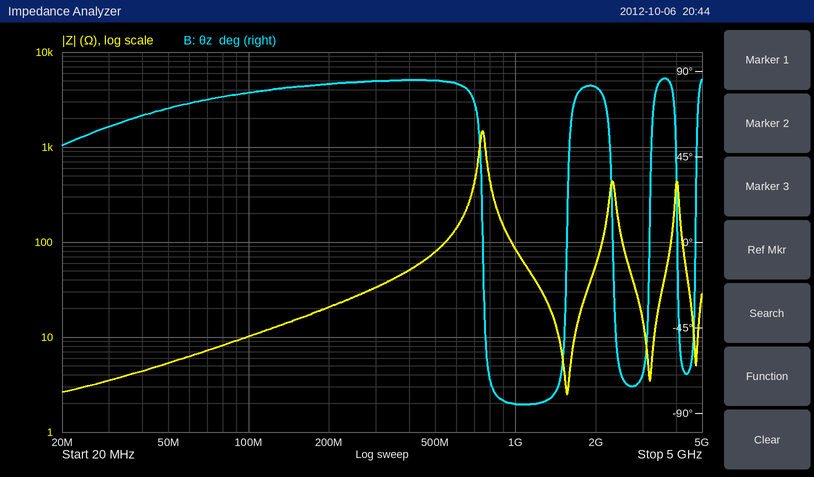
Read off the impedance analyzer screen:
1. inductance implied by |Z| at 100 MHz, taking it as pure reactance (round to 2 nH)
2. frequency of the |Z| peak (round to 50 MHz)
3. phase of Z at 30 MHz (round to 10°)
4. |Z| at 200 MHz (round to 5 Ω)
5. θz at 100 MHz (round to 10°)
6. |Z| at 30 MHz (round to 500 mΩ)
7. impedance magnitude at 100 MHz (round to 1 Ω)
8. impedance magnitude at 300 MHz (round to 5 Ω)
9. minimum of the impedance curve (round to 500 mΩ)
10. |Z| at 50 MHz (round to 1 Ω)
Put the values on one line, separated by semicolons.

16 nH; 750 MHz; 60°; 20 Ω; 80°; 3.5 Ω; 10 Ω; 35 Ω; 2.5 Ω; 5 Ω
